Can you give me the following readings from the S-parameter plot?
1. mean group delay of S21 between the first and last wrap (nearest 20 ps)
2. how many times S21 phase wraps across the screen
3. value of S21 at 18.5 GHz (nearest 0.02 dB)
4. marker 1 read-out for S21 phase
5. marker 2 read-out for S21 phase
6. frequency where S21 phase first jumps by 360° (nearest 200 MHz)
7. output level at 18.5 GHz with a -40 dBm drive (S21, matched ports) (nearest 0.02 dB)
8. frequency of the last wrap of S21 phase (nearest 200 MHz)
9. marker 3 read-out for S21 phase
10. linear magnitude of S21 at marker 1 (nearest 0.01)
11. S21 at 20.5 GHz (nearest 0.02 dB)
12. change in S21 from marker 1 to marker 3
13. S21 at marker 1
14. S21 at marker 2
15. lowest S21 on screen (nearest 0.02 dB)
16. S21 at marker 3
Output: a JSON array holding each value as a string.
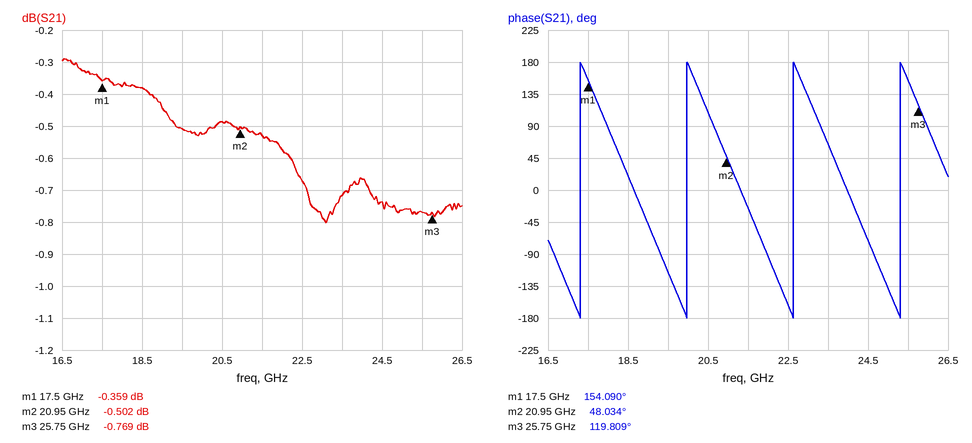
["380 ps", "4", "-0.38 dB", "154.090°", "48.034°", "17.4 GHz", "-40.38 dBm", "25.4 GHz", "119.809°", "0.96", "-0.48 dB", "-0.410 dB", "-0.359 dB", "-0.502 dB", "-0.80 dB", "-0.769 dB"]
